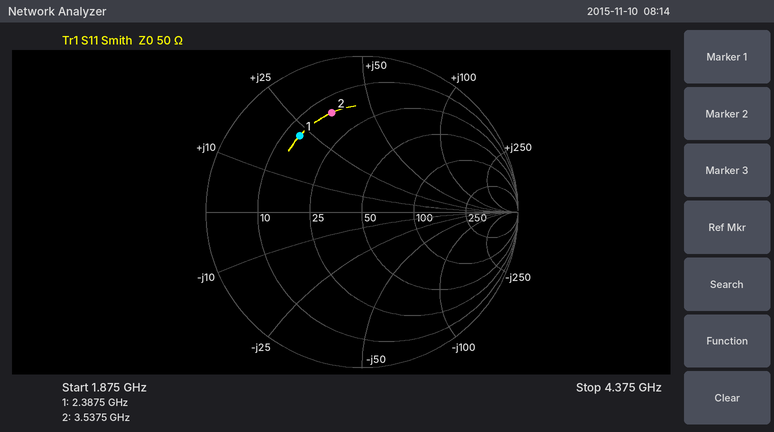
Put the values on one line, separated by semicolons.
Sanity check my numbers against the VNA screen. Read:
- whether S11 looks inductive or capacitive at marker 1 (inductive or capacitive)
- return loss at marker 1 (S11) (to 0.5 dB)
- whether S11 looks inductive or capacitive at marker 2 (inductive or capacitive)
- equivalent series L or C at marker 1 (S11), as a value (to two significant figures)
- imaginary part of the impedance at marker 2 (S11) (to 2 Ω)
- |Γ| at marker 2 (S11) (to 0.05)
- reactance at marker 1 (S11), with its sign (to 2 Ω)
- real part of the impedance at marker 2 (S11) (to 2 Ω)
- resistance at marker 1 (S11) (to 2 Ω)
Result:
inductive; 4.0 dB; inductive; 1.5 nH; +34 Ω; 0.65; +22 Ω; 16 Ω; 14 Ω
